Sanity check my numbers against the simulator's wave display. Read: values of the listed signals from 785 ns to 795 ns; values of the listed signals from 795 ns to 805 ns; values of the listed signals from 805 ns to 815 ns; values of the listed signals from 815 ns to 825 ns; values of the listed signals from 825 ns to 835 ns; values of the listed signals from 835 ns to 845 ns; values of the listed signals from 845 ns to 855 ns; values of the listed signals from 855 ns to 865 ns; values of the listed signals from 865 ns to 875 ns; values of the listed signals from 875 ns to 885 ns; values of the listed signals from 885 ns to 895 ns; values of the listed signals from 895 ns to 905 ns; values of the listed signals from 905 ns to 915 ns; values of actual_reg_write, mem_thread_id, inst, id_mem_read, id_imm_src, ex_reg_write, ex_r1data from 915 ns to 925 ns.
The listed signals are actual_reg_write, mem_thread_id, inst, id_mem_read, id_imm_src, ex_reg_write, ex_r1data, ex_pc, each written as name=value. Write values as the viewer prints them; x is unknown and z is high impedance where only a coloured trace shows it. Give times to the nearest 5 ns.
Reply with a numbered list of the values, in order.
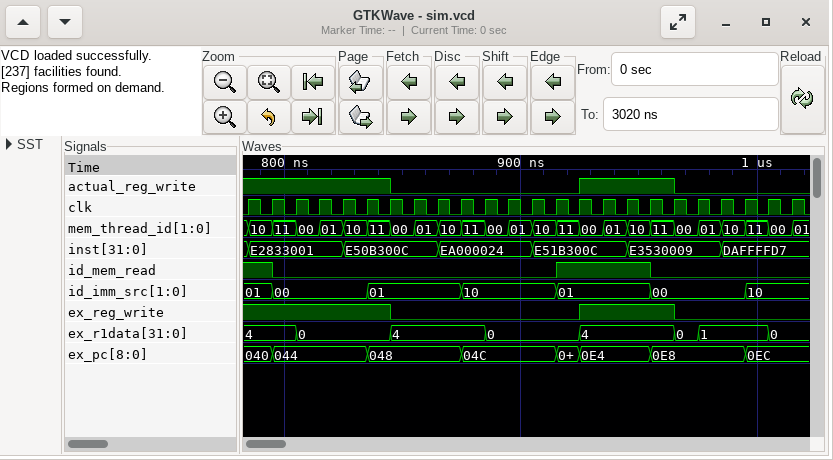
1. actual_reg_write=1, mem_thread_id=10, inst=E2833001, id_mem_read=1, id_imm_src=01, ex_reg_write=1, ex_r1data=4, ex_pc=040
2. actual_reg_write=1, mem_thread_id=11, inst=E2833001, id_mem_read=0, id_imm_src=00, ex_reg_write=1, ex_r1data=4, ex_pc=044
3. actual_reg_write=1, mem_thread_id=00, inst=E2833001, id_mem_read=0, id_imm_src=00, ex_reg_write=1, ex_r1data=0, ex_pc=044
4. actual_reg_write=1, mem_thread_id=01, inst=E2833001, id_mem_read=0, id_imm_src=00, ex_reg_write=1, ex_r1data=0, ex_pc=044
5. actual_reg_write=1, mem_thread_id=10, inst=E50B300C, id_mem_read=0, id_imm_src=00, ex_reg_write=1, ex_r1data=0, ex_pc=044
6. actual_reg_write=1, mem_thread_id=11, inst=E50B300C, id_mem_read=0, id_imm_src=01, ex_reg_write=1, ex_r1data=0, ex_pc=048
7. actual_reg_write=0, mem_thread_id=00, inst=E50B300C, id_mem_read=0, id_imm_src=01, ex_reg_write=0, ex_r1data=4, ex_pc=048
8. actual_reg_write=0, mem_thread_id=01, inst=E50B300C, id_mem_read=0, id_imm_src=01, ex_reg_write=0, ex_r1data=4, ex_pc=048
9. actual_reg_write=0, mem_thread_id=10, inst=EA000024, id_mem_read=0, id_imm_src=01, ex_reg_write=0, ex_r1data=4, ex_pc=048
10. actual_reg_write=0, mem_thread_id=11, inst=EA000024, id_mem_read=0, id_imm_src=10, ex_reg_write=0, ex_r1data=4, ex_pc=04C
11. actual_reg_write=0, mem_thread_id=00, inst=EA000024, id_mem_read=0, id_imm_src=10, ex_reg_write=0, ex_r1data=0, ex_pc=04C
12. actual_reg_write=0, mem_thread_id=01, inst=EA000024, id_mem_read=0, id_imm_src=10, ex_reg_write=0, ex_r1data=0, ex_pc=04C
13. actual_reg_write=0, mem_thread_id=10, inst=E51B300C, id_mem_read=0, id_imm_src=10, ex_reg_write=0, ex_r1data=0, ex_pc=04C
14. actual_reg_write=0, mem_thread_id=11, inst=E51B300C, id_mem_read=1, id_imm_src=01, ex_reg_write=0, ex_r1data=0
